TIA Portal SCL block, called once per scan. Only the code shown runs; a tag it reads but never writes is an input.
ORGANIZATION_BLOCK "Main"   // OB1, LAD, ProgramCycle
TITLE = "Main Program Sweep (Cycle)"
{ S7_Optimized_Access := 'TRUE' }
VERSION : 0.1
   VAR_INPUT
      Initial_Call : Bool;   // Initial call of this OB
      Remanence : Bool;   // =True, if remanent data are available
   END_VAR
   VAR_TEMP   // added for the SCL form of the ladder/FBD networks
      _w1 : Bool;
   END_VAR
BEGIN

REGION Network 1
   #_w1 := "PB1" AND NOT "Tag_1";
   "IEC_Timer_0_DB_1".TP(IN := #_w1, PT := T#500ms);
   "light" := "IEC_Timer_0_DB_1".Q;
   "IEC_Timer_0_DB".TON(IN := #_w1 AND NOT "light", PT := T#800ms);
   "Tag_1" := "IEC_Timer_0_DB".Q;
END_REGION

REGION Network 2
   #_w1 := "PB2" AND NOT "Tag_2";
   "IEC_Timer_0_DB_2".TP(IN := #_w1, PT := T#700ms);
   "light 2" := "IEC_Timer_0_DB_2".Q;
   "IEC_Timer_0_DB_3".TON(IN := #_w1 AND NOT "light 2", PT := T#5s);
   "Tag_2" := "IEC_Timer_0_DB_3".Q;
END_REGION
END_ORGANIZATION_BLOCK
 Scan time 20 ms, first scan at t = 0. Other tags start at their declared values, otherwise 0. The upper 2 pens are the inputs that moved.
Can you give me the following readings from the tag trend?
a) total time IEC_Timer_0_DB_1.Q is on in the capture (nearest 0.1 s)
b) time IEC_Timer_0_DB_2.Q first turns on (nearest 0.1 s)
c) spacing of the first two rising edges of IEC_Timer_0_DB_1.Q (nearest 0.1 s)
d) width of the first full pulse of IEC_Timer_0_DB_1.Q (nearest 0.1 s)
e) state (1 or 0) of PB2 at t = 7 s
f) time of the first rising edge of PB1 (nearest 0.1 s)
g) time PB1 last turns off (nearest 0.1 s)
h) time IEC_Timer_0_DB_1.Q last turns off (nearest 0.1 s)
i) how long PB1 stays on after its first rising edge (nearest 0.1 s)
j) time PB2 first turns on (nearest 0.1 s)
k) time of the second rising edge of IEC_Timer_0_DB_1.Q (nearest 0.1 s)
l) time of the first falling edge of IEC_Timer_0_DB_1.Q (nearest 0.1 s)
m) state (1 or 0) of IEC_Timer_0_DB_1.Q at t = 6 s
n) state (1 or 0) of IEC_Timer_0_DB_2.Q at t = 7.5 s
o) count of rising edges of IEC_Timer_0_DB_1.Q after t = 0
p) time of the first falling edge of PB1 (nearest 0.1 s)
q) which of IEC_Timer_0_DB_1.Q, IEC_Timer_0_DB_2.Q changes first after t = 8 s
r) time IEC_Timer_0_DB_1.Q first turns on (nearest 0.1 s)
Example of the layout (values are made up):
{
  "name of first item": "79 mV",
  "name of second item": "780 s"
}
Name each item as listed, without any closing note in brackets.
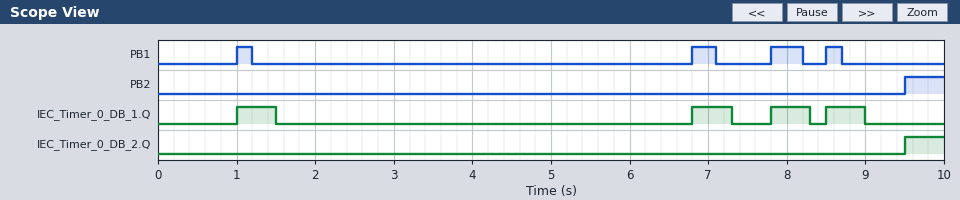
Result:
{
  "total time IEC_Timer_0_DB_1.Q is on in the capture": "2.0 s",
  "time IEC_Timer_0_DB_2.Q first turns on": "9.5 s",
  "spacing of the first two rising edges of IEC_Timer_0_DB_1.Q": "5.8 s",
  "width of the first full pulse of IEC_Timer_0_DB_1.Q": "0.5 s",
  "state (1 or 0) of PB2 at t = 7 s": "0",
  "time of the first rising edge of PB1": "1.0 s",
  "time PB1 last turns off": "8.7 s",
  "time IEC_Timer_0_DB_1.Q last turns off": "9.0 s",
  "how long PB1 stays on after its first rising edge": "0.2 s",
  "time PB2 first turns on": "9.5 s",
  "time of the second rising edge of IEC_Timer_0_DB_1.Q": "6.8 s",
  "time of the first falling edge of IEC_Timer_0_DB_1.Q": "1.5 s",
  "state (1 or 0) of IEC_Timer_0_DB_1.Q at t = 6 s": "0",
  "state (1 or 0) of IEC_Timer_0_DB_2.Q at t = 7.5 s": "0",
  "count of rising edges of IEC_Timer_0_DB_1.Q after t = 0": "4",
  "time of the first falling edge of PB1": "1.2 s",
  "which of IEC_Timer_0_DB_1.Q, IEC_Timer_0_DB_2.Q changes first after t = 8 s": "IEC_Timer_0_DB_1.Q",
  "time IEC_Timer_0_DB_1.Q first turns on": "1.0 s"
}
